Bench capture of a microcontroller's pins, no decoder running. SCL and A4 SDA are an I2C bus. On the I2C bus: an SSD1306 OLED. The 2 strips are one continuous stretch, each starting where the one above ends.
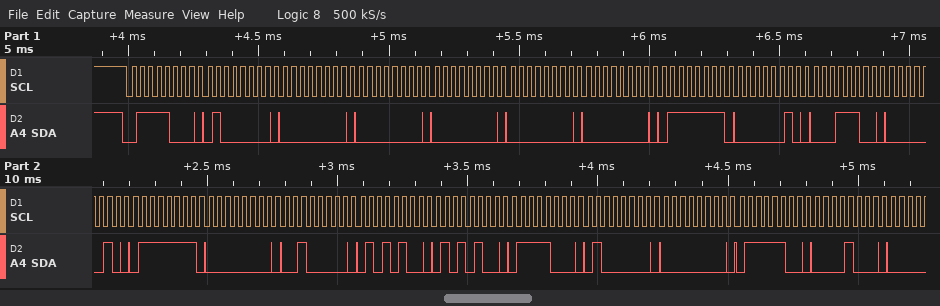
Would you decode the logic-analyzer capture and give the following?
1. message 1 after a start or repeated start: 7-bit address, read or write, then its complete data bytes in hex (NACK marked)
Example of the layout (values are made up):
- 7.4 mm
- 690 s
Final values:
- 0x3C write: 40 00 00 00 00 00 7F 02 1C 02 7F 00 20 54 54 78 40 00 7C 08
